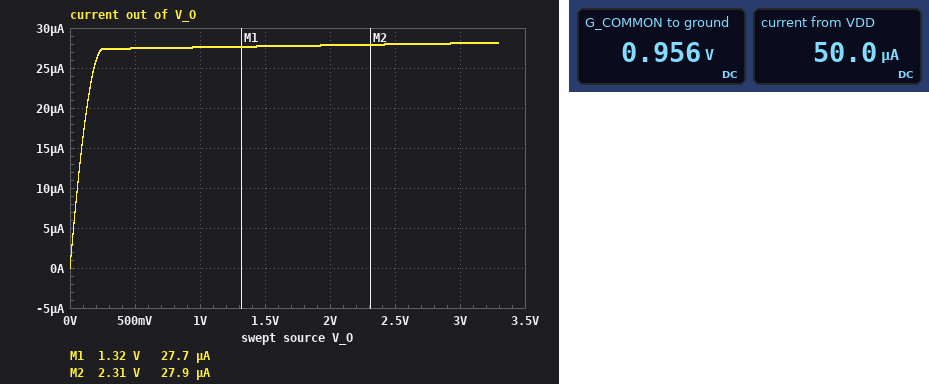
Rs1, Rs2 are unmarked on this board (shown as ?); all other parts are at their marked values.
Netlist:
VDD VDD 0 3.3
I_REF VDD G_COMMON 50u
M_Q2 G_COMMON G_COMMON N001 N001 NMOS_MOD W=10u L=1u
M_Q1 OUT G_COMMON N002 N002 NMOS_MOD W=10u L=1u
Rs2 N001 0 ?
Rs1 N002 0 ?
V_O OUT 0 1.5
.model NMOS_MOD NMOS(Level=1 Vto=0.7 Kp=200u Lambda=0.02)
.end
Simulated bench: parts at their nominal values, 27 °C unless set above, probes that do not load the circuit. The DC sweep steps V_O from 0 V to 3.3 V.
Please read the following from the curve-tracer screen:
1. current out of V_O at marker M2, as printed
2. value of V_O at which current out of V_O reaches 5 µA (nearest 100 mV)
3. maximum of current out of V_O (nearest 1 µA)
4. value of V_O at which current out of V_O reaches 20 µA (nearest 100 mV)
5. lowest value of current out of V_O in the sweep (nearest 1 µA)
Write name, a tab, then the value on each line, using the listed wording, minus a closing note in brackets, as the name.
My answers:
current out of V_O at marker M2, as printed	27.9 µA
value of V_O at which current out of V_O reaches 5 µA	0 V
maximum of current out of V_O	28 µA
value of V_O at which current out of V_O reaches 20 µA	100 mV
lowest value of current out of V_O in the sweep	0 A
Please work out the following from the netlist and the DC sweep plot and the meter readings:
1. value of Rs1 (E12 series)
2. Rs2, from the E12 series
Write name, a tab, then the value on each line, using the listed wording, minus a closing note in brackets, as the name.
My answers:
value of Rs1	3.3 kΩ
Rs2, from the E12 series	680 Ω
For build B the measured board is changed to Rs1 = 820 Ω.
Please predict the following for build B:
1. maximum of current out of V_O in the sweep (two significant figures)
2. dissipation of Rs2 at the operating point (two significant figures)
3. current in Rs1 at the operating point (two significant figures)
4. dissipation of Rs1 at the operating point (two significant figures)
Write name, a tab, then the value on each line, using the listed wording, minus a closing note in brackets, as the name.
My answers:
maximum of current out of V_O in the sweep	49 µA
dissipation of Rs2 at the operating point	1.7 µW
current in Rs1 at the operating point	48 µA
dissipation of Rs1 at the operating point	1.9 µW
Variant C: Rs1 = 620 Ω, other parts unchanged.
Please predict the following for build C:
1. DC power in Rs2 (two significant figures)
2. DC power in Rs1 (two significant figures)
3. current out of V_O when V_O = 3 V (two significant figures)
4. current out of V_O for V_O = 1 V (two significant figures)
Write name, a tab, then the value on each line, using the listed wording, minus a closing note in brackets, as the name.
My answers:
DC power in Rs2	1.7 µW
DC power in Rs1	1.6 µW
current out of V_O when V_O = 3 V	53 µA
current out of V_O for V_O = 1 V	51 µA
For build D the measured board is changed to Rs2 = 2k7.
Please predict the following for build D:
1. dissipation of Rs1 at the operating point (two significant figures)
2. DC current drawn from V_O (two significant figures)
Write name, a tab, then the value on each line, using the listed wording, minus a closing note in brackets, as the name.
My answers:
dissipation of Rs1 at the operating point	6.6 µW
DC current drawn from V_O	45 µA
